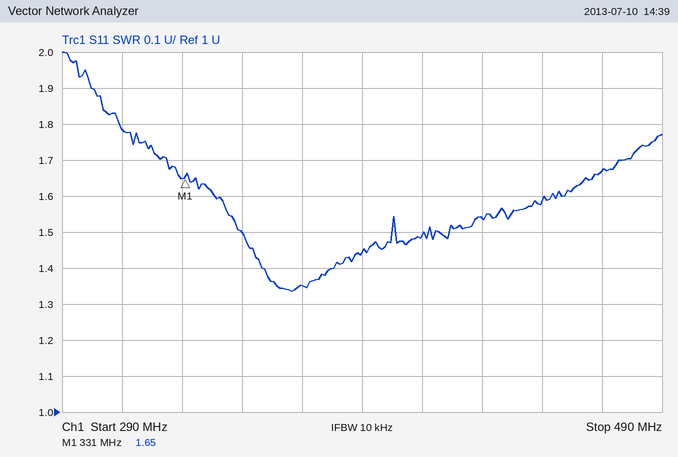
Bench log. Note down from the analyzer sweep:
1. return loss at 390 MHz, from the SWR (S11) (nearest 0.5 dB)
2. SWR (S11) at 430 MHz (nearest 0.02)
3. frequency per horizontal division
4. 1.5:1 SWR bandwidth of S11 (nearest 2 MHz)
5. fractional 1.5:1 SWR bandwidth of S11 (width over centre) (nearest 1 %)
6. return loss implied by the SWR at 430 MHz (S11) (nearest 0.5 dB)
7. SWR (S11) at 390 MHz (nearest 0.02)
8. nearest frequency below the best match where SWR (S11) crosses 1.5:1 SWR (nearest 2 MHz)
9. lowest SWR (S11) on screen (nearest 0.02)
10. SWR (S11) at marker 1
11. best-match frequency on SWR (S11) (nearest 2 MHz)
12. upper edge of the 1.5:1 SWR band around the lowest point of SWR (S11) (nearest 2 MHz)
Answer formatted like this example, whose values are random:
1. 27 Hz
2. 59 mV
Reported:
1. 15.0 dB
2. 1.54
3. 20 MHz
4. 50 MHz
5. 13 %
6. 13.5 dB
7. 1.44
8. 350 MHz
9. 1.34
10. 1.65
11. 366 MHz
12. 400 MHz
